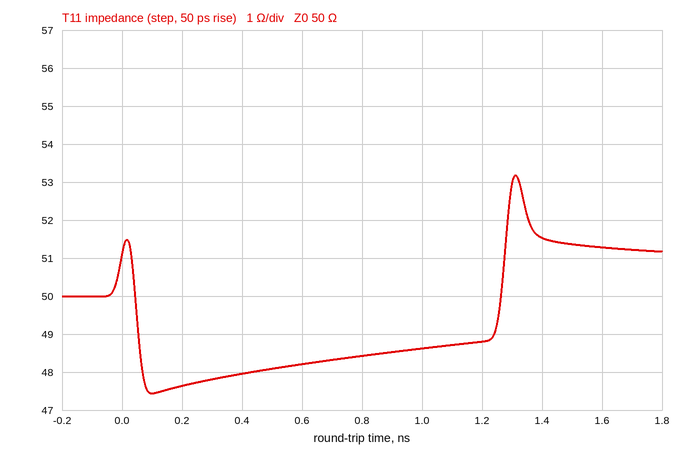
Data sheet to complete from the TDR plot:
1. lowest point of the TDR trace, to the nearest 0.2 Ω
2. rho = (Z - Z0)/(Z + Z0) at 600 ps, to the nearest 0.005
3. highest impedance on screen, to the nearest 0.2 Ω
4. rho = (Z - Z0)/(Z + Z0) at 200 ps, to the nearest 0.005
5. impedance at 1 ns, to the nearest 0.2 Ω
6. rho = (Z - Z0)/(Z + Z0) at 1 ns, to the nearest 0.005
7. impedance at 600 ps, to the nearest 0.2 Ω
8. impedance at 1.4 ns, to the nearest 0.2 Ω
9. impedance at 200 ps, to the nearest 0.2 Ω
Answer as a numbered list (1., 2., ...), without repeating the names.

1. 47.4 Ω
2. -0.020
3. 53.2 Ω
4. -0.025
5. 48.6 Ω
6. -0.015
7. 48.2 Ω
8. 51.6 Ω
9. 47.6 Ω
